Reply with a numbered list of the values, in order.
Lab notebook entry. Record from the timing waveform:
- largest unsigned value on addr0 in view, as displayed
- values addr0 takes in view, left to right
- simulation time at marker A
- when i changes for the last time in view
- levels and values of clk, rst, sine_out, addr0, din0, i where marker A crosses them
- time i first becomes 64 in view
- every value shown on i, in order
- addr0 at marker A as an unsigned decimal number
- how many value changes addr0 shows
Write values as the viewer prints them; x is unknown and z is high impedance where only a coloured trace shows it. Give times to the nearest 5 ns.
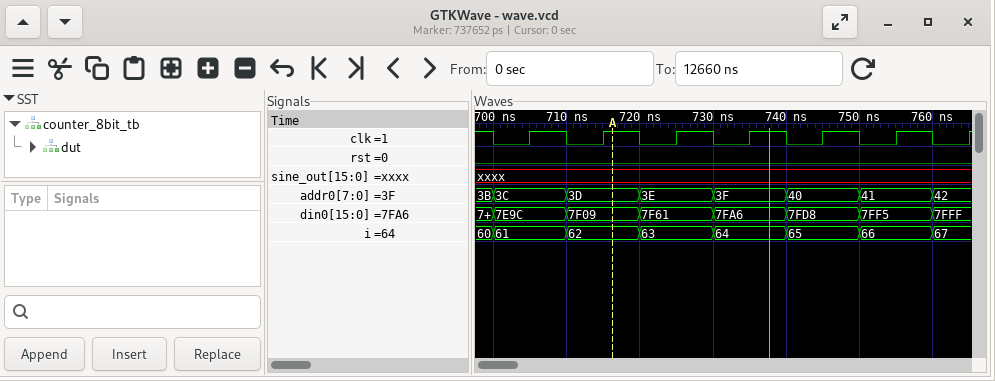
1. 42
2. 3B, 3C, 3D, 3E, 3F, 40, 41, 42
3. 715 ns
4. 760 ns
5. clk=1, rst=0, sine_out=xxxx, addr0=3D, din0=7F09, i=62
6. 730 ns
7. 60, 61, 62, 63, 64, 65, 66, 67
8. 61
9. 7
